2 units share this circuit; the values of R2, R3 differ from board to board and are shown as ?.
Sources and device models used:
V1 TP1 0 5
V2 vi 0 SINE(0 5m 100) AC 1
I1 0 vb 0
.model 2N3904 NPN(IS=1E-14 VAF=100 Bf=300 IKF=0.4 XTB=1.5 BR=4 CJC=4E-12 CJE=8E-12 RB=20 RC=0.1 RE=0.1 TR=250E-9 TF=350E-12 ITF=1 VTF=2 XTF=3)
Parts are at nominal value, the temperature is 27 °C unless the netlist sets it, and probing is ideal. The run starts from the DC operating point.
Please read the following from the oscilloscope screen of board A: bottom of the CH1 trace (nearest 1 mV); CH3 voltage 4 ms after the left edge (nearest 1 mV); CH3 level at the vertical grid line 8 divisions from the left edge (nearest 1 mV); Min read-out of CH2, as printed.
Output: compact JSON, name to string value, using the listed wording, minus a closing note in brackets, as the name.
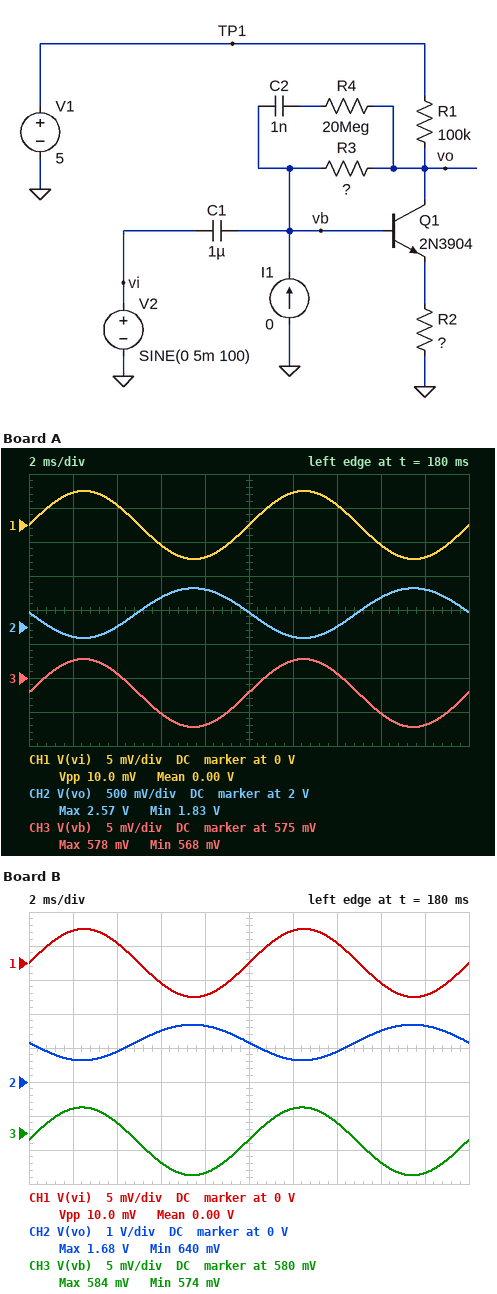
{"bottom of the CH1 trace": "-5 mV", "CH3 voltage 4 ms after the left edge": "576 mV", "CH3 level at the vertical grid line 8 divisions from the left edge": "570 mV", "Min read-out of CH2, as printed": "1.83 V"}
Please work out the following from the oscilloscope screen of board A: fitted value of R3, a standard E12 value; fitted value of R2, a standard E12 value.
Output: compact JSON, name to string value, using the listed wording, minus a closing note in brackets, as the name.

{"fitted value of R3, a standard E12 value": "18 MΩ", "fitted value of R2, a standard E12 value": "390 Ω"}
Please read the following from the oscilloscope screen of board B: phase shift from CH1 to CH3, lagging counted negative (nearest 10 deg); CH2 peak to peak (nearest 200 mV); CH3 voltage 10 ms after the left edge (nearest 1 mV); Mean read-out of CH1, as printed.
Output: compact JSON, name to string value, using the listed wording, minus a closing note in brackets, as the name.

{"phase shift from CH1 to CH3, lagging counted negative": "0 deg", "CH2 peak to peak": "1.0 V", "CH3 voltage 10 ms after the left edge": "579 mV", "Mean read-out of CH1, as printed": "0.00 V"}
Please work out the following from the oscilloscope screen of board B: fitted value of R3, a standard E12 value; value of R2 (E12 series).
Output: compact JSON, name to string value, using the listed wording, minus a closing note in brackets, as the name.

{"fitted value of R3, a standard E12 value": "4.7 MΩ", "value of R2": "220 Ω"}
